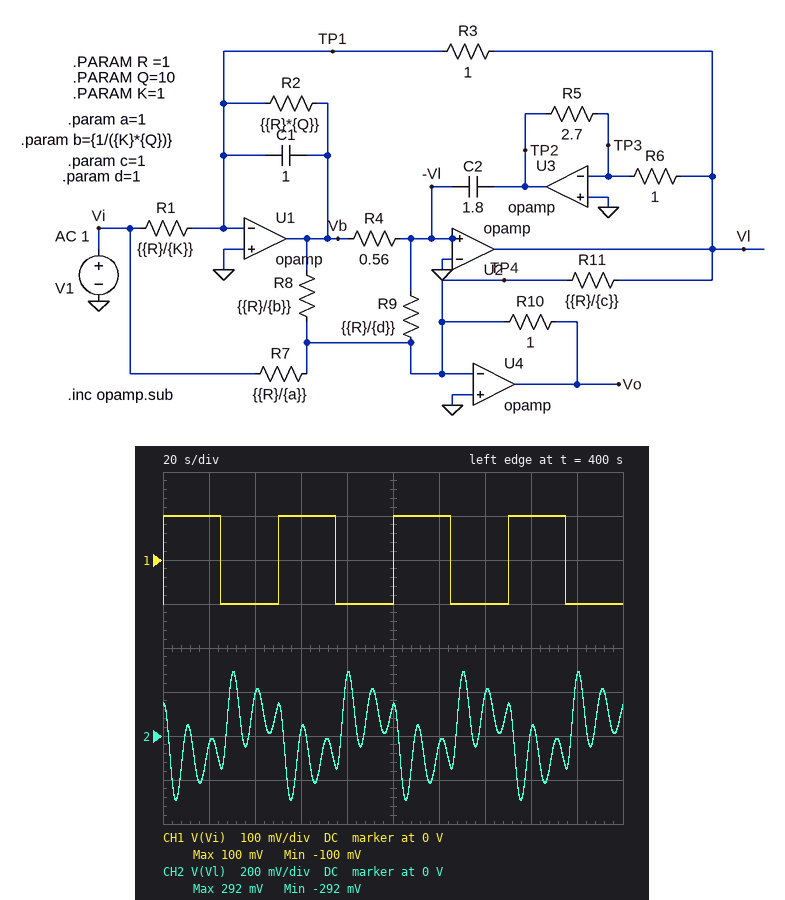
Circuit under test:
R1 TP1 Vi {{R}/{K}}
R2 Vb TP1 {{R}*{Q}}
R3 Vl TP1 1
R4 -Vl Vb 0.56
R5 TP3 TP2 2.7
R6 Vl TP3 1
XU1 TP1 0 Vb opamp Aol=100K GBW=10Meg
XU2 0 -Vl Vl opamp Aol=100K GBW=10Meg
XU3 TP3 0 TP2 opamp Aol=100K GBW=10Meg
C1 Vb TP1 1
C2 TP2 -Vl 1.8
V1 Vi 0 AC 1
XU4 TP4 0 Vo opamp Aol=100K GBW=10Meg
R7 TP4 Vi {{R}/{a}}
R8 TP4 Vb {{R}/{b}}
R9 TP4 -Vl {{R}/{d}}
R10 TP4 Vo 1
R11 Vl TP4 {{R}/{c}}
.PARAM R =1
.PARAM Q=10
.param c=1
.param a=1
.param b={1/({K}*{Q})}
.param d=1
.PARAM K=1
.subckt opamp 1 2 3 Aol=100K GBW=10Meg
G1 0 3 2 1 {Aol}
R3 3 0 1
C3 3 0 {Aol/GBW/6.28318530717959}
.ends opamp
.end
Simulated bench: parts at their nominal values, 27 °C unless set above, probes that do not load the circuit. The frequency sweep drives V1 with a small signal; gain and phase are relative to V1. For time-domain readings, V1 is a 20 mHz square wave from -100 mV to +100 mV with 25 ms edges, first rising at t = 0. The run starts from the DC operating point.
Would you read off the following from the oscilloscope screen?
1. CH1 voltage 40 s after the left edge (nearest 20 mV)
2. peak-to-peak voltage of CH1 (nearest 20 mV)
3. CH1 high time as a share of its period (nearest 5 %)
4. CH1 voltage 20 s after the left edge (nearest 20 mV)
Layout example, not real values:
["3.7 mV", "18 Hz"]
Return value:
["-100 mV", "200 mV", "50 %", "100 mV"]
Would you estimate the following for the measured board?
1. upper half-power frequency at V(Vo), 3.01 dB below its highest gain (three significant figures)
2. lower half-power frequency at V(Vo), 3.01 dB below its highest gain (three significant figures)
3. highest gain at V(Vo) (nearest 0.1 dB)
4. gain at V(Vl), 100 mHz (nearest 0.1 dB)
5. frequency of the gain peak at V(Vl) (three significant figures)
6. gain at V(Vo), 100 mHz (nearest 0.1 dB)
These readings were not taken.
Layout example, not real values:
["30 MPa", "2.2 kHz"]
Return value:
["106 mHz", "89.9 mHz", "15.7 dB", "14.6 dB", "95.8 mHz", "15.2 dB"]
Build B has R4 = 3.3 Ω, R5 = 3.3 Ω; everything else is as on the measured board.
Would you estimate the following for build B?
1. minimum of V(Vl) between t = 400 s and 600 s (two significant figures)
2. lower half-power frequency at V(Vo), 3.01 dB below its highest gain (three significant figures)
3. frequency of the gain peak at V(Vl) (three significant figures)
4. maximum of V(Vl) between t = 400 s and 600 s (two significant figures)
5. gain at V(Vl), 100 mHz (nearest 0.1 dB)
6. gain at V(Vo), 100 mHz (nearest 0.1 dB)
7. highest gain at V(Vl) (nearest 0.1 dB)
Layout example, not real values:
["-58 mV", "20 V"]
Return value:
["-180 mV", "31.1 mHz", "34.1 mHz", "180 mV", "-16.7 dB", "1.1 dB", "7.3 dB"]
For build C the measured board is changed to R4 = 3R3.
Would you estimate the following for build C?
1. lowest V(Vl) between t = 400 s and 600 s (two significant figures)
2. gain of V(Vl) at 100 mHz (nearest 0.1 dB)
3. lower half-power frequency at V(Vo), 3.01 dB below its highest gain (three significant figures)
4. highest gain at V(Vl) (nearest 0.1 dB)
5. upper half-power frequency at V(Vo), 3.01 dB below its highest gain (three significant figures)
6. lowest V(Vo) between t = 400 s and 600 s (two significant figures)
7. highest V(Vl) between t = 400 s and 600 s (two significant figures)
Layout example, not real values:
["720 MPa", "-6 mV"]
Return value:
["-180 mV", "-14.7 dB", "34.7 mHz", "8.1 dB", "54.7 mHz", "-150 mV", "180 mV"]
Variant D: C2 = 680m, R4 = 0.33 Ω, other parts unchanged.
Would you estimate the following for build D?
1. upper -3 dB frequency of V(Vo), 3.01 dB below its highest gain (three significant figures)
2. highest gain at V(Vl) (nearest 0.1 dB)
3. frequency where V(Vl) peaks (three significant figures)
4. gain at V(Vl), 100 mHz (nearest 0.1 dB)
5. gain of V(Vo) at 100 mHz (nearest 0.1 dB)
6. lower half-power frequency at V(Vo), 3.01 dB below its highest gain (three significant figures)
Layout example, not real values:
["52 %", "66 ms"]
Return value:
["213 mHz", "22.2 dB", "204 mHz", "2.4 dB", "-10.1 dB", "197 mHz"]
